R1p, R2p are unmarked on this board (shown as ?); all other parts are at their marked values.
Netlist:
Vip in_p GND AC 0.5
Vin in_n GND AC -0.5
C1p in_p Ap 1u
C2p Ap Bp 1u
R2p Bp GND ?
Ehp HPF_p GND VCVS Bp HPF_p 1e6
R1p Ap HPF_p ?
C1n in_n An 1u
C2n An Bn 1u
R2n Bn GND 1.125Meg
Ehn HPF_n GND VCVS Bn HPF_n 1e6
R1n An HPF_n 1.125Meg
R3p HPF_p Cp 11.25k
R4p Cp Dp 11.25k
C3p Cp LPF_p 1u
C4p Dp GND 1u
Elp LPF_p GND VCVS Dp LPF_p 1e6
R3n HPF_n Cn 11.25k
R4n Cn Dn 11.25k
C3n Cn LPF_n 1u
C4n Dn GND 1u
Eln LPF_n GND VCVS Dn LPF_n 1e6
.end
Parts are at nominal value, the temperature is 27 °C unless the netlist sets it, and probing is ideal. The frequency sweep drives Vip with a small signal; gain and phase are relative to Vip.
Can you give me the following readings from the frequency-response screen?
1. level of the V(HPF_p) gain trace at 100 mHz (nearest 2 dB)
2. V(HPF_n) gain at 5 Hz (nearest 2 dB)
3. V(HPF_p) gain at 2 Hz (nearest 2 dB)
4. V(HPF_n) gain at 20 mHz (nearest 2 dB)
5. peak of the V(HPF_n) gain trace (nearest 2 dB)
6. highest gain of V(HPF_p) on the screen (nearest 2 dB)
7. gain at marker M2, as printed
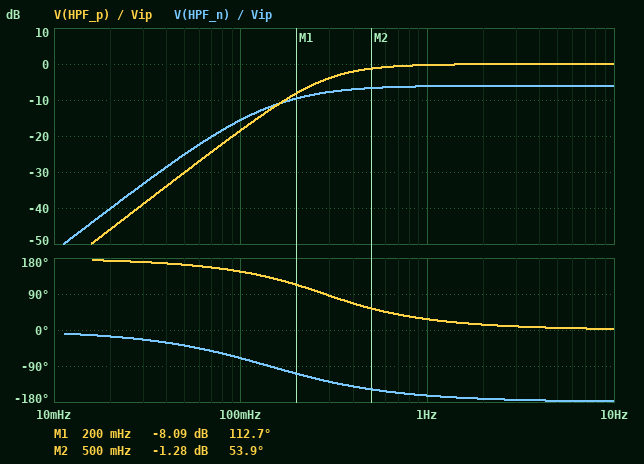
-18 dB
-6 dB
0 dB
-40 dB
-6 dB
0 dB
-1.28 dB
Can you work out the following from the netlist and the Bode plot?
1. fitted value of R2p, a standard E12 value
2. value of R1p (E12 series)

680 kΩ
470 kΩ
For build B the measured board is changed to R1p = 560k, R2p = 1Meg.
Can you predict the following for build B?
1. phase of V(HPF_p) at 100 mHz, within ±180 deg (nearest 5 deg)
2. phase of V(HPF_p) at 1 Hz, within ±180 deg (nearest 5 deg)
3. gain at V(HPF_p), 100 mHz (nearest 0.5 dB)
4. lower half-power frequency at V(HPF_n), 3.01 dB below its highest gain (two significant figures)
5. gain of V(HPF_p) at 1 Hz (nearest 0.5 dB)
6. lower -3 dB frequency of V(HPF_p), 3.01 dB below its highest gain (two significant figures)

140 deg
20 deg
-13.5 dB
220 mHz
0 dB
230 mHz
